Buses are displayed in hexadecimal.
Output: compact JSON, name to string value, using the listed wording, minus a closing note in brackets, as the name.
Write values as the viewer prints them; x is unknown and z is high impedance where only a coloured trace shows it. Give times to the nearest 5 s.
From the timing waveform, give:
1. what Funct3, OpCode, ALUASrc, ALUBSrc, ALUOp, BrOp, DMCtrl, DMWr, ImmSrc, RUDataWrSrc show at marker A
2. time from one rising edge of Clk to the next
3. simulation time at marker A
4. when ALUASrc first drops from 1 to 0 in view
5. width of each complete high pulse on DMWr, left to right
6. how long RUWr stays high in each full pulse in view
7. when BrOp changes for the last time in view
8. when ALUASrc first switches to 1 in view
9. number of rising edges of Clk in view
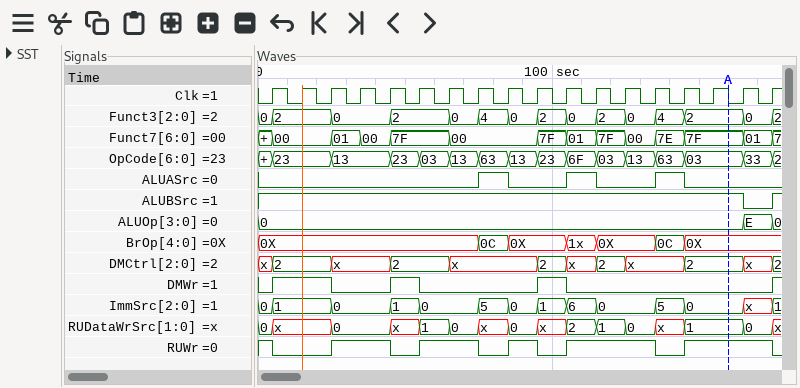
{"what Funct3, OpCode, ALUASrc, ALUBSrc, ALUOp, BrOp, DMCtrl, DMWr, ImmSrc, RUDataWrSrc show at marker A": "Funct3=2, OpCode=03, ALUASrc=0, ALUBSrc=1, ALUOp=0, BrOp=0X, DMCtrl=2, DMWr=0, ImmSrc=0, RUDataWrSrc=1", "time from one rising edge of Clk to the next": "10 s", "simulation time at marker A": "160 s", "when ALUASrc first drops from 1 to 0 in view": "85 s", "width of each complete high pulse on DMWr, left to right": "20 s, 10 s, 10 s", "how long RUWr stays high in each full pulse in view": "20 s, 20 s, 10 s, 30 s, 30 s", "when BrOp changes for the last time in view": "145 s", "when ALUASrc first switches to 1 in view": "75 s", "number of rising edges of Clk in view": "18"}
